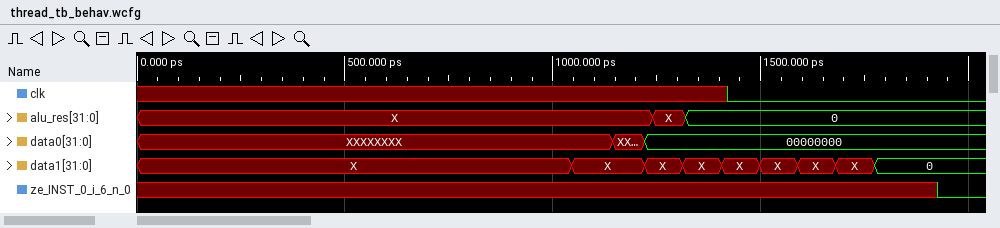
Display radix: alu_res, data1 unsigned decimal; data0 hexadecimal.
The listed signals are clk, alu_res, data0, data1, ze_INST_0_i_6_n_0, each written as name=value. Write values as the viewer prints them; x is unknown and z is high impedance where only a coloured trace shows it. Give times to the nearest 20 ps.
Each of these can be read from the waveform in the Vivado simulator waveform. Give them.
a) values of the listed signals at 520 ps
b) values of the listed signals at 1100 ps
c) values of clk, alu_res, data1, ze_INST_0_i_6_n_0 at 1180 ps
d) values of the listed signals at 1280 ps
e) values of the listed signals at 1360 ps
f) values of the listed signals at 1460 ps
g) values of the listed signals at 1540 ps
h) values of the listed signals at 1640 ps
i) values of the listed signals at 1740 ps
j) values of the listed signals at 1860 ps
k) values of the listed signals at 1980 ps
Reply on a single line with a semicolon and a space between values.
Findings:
clk=x, alu_res=X, data0=XXXXXXXX, data1=X, ze_INST_0_i_6_n_0=x; clk=x, alu_res=X, data0=XXXXXXXX, data1=X, ze_INST_0_i_6_n_0=x; clk=x, alu_res=X, data1=X, ze_INST_0_i_6_n_0=x; clk=x, alu_res=X, data0=00000000, data1=X, ze_INST_0_i_6_n_0=x; clk=x, alu_res=0, data0=00000000, data1=X, ze_INST_0_i_6_n_0=x; clk=0, alu_res=0, data0=00000000, data1=X, ze_INST_0_i_6_n_0=x; clk=0, alu_res=0, data0=00000000, data1=X, ze_INST_0_i_6_n_0=x; clk=0, alu_res=0, data0=00000000, data1=X, ze_INST_0_i_6_n_0=x; clk=0, alu_res=0, data0=00000000, data1=X, ze_INST_0_i_6_n_0=x; clk=0, alu_res=0, data0=00000000, data1=0, ze_INST_0_i_6_n_0=x; clk=0, alu_res=0, data0=00000000, data1=0, ze_INST_0_i_6_n_0=0
